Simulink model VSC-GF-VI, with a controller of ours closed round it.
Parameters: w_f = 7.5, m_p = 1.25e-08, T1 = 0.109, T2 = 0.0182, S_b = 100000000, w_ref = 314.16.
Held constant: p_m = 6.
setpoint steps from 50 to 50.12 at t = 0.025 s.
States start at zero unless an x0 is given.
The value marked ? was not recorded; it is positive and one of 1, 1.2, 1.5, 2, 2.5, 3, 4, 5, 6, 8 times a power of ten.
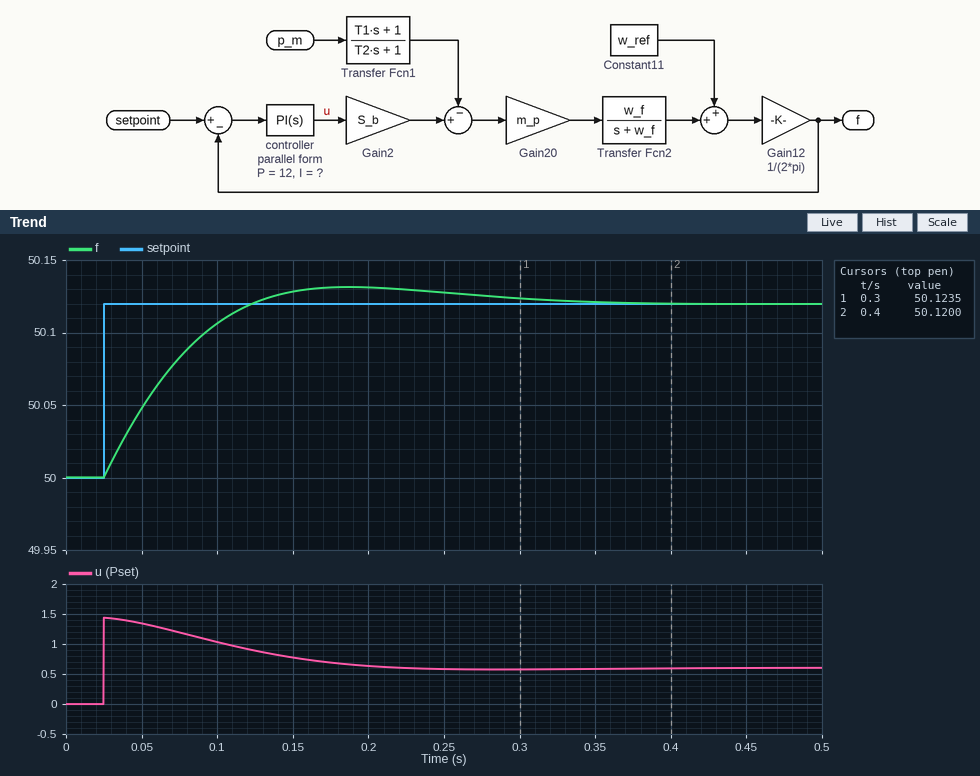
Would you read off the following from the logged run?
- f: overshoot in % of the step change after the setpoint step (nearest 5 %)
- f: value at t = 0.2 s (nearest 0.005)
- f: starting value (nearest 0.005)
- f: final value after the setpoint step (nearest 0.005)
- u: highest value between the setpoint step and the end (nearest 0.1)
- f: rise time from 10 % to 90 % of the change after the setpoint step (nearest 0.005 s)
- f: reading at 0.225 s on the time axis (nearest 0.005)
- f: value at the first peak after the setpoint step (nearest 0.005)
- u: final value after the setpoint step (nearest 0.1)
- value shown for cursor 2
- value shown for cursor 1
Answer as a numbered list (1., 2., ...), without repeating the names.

1. 10 %
2. 50.130
3. 50.000
4. 50.120
5. 1.4
6. 0.070 s
7. 50.130
8. 50.130
9. 0.6
10. 50.1200
11. 50.1235
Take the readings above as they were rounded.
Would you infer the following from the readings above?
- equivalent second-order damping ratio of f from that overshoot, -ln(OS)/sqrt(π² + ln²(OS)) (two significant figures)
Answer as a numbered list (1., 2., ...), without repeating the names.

1. 0.59
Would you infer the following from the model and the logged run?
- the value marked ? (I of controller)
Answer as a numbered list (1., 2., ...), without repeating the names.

1. 200
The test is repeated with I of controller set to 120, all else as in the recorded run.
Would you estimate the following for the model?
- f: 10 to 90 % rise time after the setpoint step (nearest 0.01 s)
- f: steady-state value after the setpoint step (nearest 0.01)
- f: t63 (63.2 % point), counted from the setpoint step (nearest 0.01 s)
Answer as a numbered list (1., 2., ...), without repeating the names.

1. 0.10 s
2. 50.12
3. 0.05 s
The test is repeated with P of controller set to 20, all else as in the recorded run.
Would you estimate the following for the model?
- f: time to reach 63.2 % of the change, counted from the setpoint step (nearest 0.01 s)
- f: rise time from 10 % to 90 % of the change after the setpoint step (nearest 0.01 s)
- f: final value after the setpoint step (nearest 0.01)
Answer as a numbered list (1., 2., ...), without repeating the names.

1. 0.03 s
2. 0.06 s
3. 50.12
